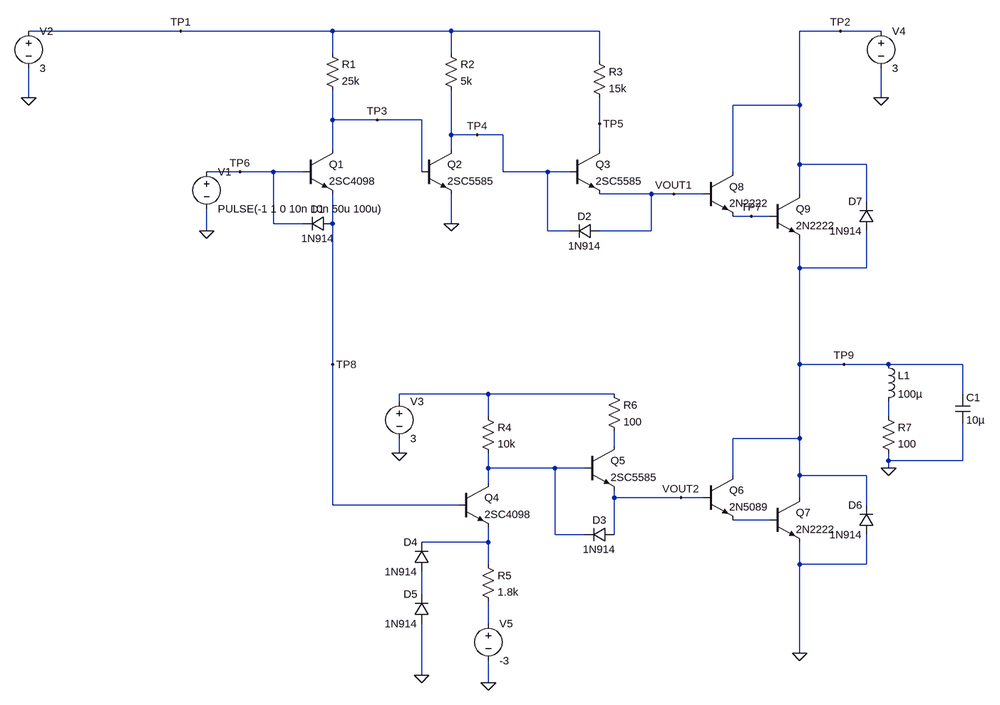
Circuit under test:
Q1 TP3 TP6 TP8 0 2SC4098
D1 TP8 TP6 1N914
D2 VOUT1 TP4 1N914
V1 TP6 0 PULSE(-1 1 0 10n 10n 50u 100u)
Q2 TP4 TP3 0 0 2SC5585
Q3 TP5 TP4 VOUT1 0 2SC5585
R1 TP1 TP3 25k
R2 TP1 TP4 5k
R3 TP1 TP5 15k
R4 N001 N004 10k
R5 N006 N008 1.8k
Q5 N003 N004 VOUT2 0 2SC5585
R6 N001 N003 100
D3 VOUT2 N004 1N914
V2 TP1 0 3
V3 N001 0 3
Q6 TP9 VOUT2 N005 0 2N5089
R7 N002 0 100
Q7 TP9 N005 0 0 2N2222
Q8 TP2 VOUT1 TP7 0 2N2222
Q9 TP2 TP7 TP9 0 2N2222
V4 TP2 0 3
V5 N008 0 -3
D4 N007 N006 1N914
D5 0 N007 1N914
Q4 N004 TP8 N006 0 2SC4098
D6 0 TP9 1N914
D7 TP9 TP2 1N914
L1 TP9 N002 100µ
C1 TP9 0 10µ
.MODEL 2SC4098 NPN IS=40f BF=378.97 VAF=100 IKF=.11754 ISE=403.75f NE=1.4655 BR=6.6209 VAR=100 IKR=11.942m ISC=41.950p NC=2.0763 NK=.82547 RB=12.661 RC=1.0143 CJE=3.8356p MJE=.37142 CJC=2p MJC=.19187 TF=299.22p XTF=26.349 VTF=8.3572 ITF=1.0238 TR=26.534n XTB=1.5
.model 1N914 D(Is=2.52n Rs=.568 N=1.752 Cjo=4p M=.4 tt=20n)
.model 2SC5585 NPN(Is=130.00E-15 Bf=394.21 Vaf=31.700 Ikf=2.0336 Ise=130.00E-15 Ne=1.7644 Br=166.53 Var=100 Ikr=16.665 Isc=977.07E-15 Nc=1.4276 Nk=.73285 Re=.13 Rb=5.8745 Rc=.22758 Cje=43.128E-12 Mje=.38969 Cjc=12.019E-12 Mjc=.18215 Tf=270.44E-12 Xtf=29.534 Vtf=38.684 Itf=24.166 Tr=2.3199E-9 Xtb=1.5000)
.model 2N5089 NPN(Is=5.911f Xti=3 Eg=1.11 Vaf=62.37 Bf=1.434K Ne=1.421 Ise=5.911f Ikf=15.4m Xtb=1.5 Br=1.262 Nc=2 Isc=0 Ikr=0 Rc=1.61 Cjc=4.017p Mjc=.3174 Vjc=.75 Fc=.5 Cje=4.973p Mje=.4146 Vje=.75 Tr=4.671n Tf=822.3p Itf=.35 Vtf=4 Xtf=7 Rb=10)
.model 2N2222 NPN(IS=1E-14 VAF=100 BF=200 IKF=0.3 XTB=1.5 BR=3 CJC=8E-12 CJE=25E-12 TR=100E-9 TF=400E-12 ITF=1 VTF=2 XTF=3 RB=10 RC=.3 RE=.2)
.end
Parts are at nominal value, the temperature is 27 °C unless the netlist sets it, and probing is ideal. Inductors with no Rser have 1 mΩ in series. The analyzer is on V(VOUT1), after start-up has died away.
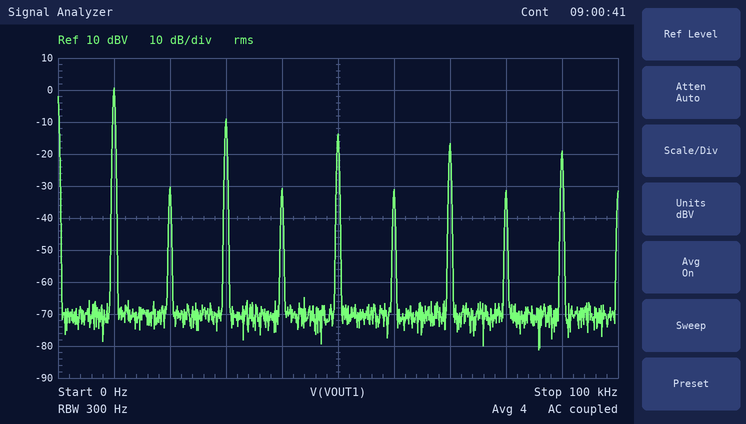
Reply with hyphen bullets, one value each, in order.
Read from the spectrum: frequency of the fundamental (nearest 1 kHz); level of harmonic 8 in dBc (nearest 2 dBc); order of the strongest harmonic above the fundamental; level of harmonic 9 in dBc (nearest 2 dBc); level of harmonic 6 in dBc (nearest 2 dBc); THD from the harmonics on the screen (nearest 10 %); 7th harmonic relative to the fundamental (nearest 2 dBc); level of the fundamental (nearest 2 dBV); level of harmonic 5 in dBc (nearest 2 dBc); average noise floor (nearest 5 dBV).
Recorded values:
- 10 kHz
- -32 dBc
- 3
- -20 dBc
- -32 dBc
- 40 %
- -18 dBc
- 0 dBV
- -14 dBc
- -70 dBV
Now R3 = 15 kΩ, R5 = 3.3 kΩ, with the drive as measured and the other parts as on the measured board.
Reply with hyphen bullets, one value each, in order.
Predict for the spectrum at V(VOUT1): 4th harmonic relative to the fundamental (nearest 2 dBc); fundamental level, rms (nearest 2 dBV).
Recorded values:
- -36 dBc
- 0 dBV
